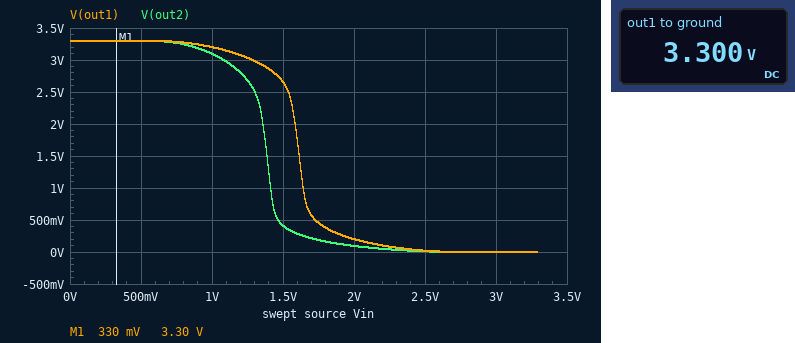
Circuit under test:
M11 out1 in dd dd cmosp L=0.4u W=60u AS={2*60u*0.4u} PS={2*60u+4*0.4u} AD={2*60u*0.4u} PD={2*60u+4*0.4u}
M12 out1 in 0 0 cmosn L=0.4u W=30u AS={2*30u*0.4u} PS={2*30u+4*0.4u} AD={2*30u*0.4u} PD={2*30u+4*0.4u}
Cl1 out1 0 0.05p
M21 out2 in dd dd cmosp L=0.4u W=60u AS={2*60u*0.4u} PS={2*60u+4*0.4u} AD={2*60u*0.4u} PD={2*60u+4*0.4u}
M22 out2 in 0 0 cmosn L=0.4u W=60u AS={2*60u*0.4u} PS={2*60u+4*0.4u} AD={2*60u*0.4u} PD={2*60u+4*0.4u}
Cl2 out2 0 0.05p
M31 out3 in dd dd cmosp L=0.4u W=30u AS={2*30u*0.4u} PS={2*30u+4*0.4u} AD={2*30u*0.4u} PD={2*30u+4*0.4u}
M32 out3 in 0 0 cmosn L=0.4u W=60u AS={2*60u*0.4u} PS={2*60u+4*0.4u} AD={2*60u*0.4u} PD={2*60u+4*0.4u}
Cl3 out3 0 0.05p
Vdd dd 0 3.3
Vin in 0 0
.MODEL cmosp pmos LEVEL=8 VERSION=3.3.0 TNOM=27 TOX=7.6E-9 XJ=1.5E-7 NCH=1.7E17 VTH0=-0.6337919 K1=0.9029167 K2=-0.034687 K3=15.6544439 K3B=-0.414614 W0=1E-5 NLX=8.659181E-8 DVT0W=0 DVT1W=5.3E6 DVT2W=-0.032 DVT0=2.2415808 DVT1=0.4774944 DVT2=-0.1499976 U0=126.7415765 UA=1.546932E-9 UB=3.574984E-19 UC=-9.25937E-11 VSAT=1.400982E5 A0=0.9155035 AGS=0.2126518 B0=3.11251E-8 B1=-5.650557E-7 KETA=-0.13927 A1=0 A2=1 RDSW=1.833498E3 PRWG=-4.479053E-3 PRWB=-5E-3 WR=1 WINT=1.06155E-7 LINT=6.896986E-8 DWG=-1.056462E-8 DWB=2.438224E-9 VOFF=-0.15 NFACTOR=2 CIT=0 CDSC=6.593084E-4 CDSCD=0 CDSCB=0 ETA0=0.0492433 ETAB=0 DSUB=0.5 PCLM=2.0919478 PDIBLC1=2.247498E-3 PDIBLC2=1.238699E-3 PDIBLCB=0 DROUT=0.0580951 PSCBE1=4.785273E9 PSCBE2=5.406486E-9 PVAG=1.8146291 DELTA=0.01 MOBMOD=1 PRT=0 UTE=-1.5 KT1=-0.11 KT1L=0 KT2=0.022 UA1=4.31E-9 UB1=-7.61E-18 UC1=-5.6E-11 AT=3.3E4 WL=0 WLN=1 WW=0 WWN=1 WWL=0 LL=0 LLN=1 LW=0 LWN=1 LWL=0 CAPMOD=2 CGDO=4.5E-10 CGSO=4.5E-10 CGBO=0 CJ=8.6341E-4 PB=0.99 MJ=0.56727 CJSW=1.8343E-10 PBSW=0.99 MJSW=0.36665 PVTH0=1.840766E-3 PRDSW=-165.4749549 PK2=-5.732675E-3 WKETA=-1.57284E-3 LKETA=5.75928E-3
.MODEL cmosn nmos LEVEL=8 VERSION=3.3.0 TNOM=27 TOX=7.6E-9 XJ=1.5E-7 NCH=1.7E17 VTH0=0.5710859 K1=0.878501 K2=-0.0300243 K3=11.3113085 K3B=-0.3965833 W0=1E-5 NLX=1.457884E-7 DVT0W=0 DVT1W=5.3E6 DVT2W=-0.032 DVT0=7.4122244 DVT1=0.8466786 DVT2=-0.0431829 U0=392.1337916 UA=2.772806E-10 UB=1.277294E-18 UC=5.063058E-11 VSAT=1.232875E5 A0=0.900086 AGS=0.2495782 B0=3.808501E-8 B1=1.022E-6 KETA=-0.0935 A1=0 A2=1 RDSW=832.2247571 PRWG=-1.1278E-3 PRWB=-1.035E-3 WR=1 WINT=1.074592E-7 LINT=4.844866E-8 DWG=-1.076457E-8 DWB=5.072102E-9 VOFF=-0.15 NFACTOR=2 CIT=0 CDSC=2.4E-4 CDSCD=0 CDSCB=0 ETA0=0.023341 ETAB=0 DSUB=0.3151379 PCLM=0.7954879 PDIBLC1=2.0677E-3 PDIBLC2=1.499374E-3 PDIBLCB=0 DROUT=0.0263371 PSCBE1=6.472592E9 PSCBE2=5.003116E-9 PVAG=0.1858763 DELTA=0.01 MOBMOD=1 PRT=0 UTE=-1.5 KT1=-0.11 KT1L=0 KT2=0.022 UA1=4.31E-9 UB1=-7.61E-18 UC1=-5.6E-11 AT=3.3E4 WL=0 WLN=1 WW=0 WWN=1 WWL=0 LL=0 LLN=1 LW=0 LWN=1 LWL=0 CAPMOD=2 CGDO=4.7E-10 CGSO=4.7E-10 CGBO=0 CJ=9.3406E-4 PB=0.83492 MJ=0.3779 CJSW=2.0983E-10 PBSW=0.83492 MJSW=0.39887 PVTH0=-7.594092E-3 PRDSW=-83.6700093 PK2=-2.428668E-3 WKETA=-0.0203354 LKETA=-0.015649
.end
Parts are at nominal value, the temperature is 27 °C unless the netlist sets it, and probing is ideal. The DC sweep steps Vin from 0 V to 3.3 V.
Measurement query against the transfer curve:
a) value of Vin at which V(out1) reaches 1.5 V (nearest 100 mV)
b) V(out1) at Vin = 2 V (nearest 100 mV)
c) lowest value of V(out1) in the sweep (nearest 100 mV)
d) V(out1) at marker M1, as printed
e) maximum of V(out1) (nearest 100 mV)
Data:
1.6 V
200 mV
0 V
3.30 V
3.3 V
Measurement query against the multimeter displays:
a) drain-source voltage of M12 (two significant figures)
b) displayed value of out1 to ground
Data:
3.3 V
3.300 V
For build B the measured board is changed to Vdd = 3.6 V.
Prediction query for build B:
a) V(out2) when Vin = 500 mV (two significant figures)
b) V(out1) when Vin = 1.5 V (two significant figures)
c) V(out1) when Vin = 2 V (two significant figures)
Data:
3.6 V
3.1 V
400 mV
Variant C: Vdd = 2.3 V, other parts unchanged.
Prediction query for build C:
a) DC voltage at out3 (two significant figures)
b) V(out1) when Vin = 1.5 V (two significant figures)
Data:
2.3 V
28 mV
